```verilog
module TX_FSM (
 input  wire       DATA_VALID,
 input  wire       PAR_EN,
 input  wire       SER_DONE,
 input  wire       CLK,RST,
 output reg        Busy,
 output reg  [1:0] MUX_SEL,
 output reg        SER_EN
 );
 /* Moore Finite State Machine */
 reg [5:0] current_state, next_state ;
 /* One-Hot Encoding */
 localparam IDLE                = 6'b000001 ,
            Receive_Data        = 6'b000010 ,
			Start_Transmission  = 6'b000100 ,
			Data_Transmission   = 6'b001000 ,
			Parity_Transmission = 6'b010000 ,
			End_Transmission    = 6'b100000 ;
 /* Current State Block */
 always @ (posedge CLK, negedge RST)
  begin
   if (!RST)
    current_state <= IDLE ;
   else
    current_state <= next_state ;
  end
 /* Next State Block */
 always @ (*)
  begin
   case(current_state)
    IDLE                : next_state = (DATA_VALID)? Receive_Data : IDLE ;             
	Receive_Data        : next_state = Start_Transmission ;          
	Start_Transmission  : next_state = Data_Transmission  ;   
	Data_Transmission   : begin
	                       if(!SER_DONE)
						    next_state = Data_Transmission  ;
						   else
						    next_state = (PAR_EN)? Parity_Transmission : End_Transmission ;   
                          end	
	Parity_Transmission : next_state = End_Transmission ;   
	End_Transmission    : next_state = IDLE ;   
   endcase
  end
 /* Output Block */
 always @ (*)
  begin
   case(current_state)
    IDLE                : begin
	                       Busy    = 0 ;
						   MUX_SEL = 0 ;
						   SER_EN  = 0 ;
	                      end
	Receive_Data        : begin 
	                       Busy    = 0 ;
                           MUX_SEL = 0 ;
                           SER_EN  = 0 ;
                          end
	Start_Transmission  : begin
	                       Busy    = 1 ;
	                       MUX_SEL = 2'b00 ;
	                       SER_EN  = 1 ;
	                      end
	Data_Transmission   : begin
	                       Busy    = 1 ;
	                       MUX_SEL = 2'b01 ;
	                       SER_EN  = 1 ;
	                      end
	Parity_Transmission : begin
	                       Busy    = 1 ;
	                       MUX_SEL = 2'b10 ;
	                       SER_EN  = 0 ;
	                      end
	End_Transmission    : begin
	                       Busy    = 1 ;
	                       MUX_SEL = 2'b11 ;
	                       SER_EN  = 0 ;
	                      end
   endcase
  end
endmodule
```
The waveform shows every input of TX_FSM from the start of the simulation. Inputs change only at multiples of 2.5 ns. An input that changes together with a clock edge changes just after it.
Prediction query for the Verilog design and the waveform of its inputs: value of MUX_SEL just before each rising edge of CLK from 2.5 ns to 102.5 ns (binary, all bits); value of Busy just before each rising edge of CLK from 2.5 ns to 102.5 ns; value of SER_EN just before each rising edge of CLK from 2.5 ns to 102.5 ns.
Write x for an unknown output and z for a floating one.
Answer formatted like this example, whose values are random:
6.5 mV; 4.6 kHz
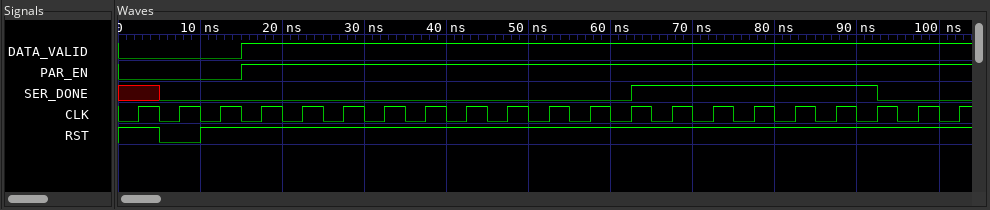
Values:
x, 00, 00, 00, 00, 00, 01, 01, 01, 01, 01, 01, 01, 01, 10, 11, 00, 00, 00, 01, 01; x 0 0 0 0 1 1 1 1 1 1 1 1 1 1 1 0 0 1 1 1; x 0 0 0 0 1 1 1 1 1 1 1 1 1 0 0 0 0 1 1 1
